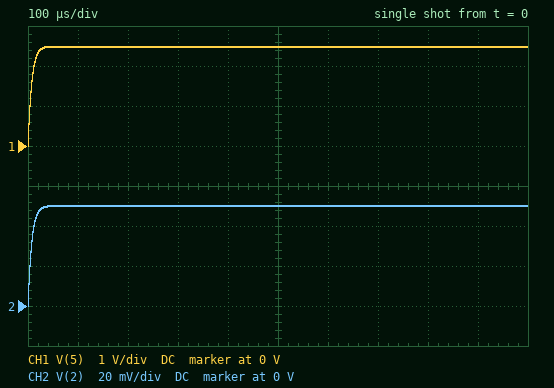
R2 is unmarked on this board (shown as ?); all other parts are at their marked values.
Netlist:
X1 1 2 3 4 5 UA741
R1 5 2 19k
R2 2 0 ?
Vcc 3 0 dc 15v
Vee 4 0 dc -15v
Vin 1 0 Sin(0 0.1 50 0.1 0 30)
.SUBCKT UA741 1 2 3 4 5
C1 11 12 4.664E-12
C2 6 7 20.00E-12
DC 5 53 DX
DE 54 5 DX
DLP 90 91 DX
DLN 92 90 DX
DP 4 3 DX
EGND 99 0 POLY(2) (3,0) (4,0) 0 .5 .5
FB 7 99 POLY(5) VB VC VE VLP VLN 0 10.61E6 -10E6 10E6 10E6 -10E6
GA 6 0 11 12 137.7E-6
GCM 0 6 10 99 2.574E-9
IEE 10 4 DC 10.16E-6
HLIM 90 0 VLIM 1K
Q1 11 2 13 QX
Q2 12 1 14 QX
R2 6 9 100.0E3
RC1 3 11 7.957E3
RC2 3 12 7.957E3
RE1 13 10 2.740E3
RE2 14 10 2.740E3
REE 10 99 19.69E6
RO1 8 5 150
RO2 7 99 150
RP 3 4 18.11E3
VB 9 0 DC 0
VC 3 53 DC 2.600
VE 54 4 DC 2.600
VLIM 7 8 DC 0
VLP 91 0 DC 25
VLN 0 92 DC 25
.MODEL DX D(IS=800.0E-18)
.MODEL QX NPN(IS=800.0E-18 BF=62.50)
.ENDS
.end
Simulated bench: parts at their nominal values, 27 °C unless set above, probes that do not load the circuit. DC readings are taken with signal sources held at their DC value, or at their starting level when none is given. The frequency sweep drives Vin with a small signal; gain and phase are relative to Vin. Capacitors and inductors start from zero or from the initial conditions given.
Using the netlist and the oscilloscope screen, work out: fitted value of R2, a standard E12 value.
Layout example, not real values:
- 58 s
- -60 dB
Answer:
- 390 Ω
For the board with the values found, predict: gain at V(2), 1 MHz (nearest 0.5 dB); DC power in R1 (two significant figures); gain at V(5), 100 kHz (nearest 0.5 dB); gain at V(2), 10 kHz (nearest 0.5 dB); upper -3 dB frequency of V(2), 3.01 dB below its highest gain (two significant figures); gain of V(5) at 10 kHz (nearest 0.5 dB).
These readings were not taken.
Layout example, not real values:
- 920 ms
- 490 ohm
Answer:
- -34.0 dB
- 310 µW
- 20.5 dB
- -1.0 dB
- 22 kHz
- 33.0 dB
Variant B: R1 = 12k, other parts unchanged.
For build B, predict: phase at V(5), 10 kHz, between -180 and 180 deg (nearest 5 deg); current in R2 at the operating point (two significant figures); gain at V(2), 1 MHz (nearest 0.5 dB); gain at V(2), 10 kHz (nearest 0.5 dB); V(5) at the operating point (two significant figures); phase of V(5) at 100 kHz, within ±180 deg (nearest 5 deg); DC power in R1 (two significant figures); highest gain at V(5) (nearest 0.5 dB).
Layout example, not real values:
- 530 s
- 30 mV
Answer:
- -15 deg
- 130 µA
- -30.0 dB
- -0.5 dB
- 1.6 V
- -75 deg
- 200 µW
- 30.0 dB
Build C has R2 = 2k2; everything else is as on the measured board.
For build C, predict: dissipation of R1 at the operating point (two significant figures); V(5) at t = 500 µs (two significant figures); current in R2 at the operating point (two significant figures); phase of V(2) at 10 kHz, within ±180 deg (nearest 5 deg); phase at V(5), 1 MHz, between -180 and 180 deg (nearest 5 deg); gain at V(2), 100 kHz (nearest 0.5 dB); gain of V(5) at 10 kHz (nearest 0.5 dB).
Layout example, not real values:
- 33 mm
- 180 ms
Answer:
- 9.9 µW
- 480 mV
- 23 µA
- -5 deg
- -110 deg
- -2.5 dB
- 19.5 dB
